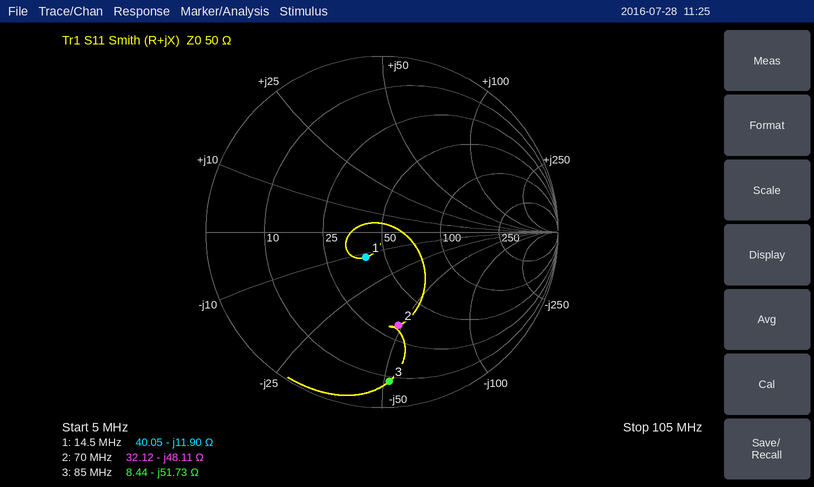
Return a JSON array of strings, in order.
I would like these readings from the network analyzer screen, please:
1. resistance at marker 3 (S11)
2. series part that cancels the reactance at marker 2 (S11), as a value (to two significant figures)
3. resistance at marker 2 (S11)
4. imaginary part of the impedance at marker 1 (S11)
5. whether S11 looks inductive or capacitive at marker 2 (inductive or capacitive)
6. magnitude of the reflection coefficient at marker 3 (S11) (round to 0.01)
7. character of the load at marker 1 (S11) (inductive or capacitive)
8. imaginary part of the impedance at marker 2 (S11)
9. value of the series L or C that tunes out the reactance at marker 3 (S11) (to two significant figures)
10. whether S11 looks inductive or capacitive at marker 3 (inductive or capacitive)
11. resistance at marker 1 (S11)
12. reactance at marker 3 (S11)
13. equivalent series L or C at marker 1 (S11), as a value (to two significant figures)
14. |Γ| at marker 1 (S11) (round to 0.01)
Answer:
["8.44 Ω", "110 nH", "32.12 Ω", "-11.90 Ω", "capacitive", "0.85", "capacitive", "-48.11 Ω", "97 nH", "capacitive", "40.05 Ω", "-51.73 Ω", "920 pF", "0.17"]
